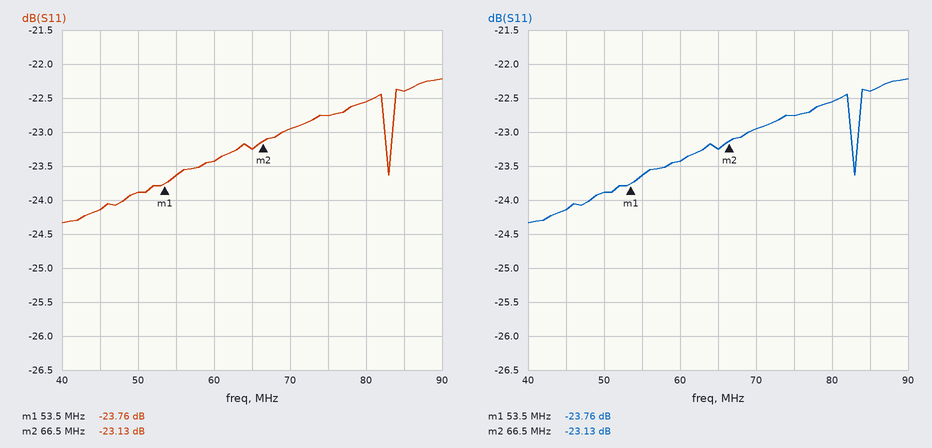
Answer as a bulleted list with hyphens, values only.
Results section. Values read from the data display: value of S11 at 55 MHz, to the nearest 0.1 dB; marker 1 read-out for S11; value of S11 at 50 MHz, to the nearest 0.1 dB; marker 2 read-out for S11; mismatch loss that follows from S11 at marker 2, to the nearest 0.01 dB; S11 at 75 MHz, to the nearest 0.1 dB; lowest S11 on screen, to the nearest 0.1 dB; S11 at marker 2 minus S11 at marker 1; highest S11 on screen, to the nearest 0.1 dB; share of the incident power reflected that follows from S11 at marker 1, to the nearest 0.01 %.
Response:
- -23.6 dB
- -23.76 dB
- -23.9 dB
- -23.13 dB
- 0.02 dB
- -22.8 dB
- -24.3 dB
- 0.63 dB
- -22.2 dB
- 0.42 %
